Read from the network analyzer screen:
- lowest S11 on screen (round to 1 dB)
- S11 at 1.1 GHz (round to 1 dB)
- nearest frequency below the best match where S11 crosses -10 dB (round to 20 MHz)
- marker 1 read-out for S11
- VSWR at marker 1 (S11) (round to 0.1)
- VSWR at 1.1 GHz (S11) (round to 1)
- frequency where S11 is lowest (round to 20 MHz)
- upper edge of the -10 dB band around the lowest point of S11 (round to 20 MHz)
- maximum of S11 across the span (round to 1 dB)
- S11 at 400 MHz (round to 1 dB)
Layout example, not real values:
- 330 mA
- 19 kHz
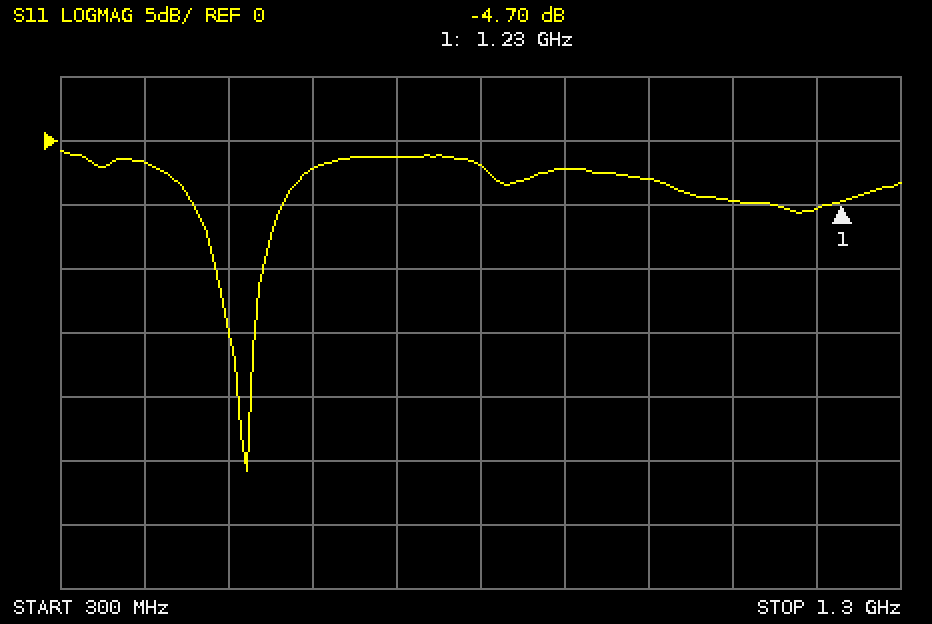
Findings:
- -26 dB
- -5 dB
- 480 MHz
- -4.70 dB
- 3.8
- 4
- 520 MHz
- 540 MHz
- -1 dB
- -2 dB
